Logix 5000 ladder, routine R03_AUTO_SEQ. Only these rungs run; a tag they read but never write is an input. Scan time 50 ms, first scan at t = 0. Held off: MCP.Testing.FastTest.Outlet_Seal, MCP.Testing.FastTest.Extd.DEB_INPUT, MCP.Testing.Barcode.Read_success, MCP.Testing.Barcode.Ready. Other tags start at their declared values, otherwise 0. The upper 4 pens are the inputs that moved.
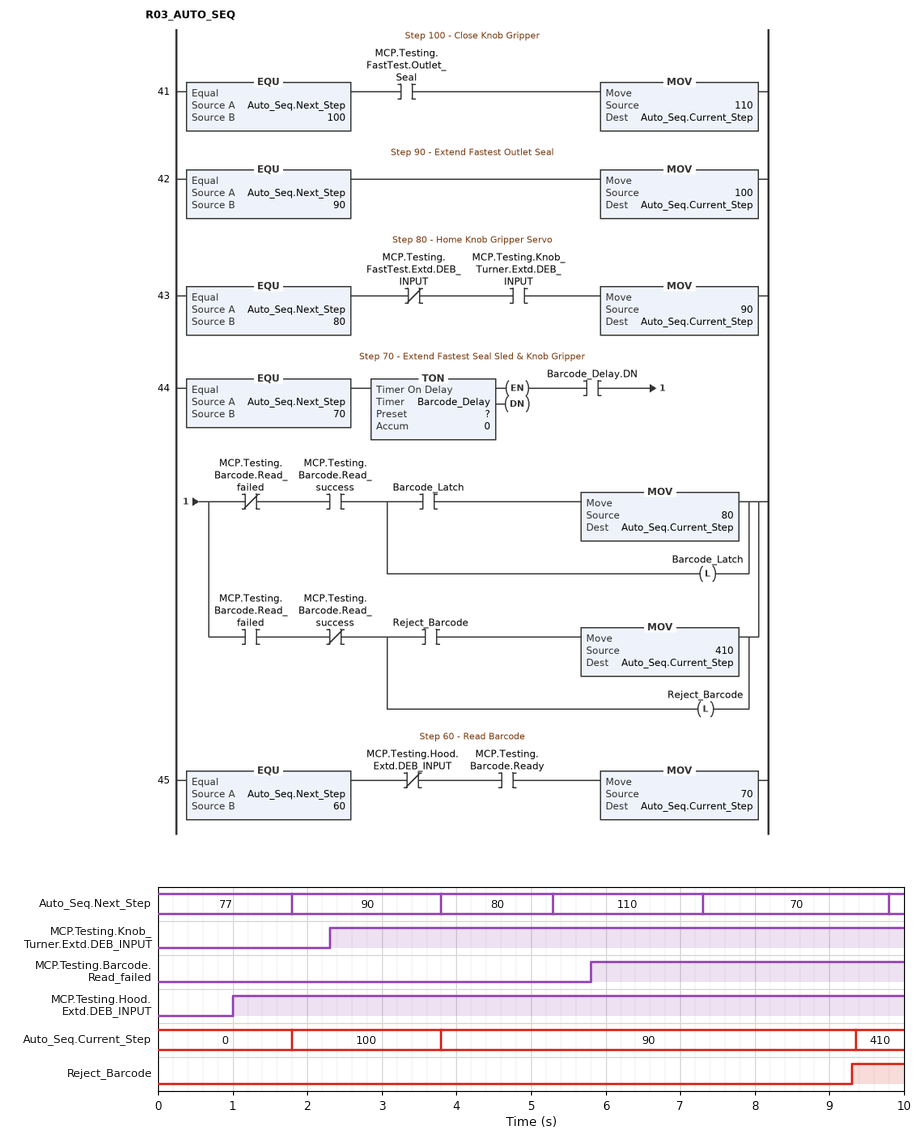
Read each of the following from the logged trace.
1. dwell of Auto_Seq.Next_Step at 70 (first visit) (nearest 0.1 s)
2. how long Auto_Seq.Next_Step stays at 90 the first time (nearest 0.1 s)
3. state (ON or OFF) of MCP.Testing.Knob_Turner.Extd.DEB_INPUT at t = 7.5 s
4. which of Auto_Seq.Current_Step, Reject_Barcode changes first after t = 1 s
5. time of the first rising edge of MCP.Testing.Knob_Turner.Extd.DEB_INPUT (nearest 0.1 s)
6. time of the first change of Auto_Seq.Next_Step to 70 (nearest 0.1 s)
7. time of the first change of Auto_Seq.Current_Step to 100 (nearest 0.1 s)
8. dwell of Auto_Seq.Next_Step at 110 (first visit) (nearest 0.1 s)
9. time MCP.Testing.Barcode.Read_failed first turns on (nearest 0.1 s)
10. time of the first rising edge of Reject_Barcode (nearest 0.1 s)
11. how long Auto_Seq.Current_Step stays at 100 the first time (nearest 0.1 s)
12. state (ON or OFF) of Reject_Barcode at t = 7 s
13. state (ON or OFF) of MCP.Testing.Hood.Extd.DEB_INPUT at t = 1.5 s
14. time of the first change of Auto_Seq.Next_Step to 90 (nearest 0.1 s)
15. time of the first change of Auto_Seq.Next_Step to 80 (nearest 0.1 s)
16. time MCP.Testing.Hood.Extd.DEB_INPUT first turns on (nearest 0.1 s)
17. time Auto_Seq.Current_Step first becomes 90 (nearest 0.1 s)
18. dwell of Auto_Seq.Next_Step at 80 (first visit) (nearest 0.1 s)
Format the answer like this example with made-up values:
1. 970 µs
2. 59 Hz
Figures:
1. 2.5 s
2. 2.0 s
3. ON
4. Auto_Seq.Current_Step
5. 2.3 s
6. 7.3 s
7. 1.8 s
8. 2.0 s
9. 5.8 s
10. 9.3 s
11. 2.0 s
12. OFF
13. ON
14. 1.8 s
15. 3.8 s
16. 1.0 s
17. 3.8 s
18. 1.5 s
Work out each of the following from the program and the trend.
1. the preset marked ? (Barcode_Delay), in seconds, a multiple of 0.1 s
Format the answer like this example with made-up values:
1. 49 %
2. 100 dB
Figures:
1. 2.0 s
